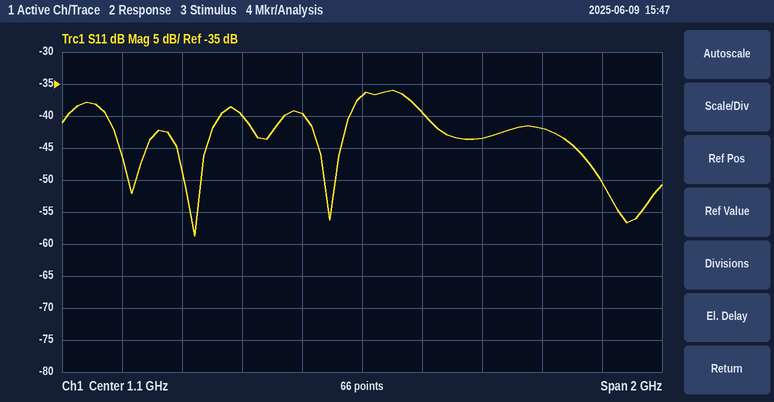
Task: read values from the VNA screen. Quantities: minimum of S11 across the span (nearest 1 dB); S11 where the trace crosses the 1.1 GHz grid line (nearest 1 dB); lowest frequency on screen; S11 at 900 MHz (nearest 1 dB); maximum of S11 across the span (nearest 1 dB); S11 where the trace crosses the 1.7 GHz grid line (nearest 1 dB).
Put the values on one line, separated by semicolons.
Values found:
-59 dB; -37 dB; 100 MHz; -40 dB; -36 dB; -42 dB
